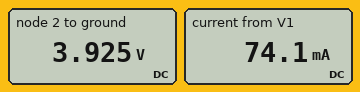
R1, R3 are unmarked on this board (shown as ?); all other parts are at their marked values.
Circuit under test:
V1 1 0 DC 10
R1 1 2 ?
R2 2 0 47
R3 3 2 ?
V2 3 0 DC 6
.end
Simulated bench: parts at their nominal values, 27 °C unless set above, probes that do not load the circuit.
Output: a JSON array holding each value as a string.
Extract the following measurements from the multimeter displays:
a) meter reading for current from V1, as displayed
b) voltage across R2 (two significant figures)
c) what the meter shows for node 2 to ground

["74.1 mA", "3.9 V", "3.925 V"]
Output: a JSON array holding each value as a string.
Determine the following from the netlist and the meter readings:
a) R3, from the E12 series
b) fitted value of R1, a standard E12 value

["220 Ω", "82 Ω"]
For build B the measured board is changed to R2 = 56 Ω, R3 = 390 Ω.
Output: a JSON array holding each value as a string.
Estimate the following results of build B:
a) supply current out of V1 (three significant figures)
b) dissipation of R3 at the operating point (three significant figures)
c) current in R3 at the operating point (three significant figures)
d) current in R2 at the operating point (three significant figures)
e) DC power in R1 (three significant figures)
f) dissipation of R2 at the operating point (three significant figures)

["70.6 mA", "8.21 mW", "4.59 mA", "75.2 mA", "409 mW", "317 mW"]
